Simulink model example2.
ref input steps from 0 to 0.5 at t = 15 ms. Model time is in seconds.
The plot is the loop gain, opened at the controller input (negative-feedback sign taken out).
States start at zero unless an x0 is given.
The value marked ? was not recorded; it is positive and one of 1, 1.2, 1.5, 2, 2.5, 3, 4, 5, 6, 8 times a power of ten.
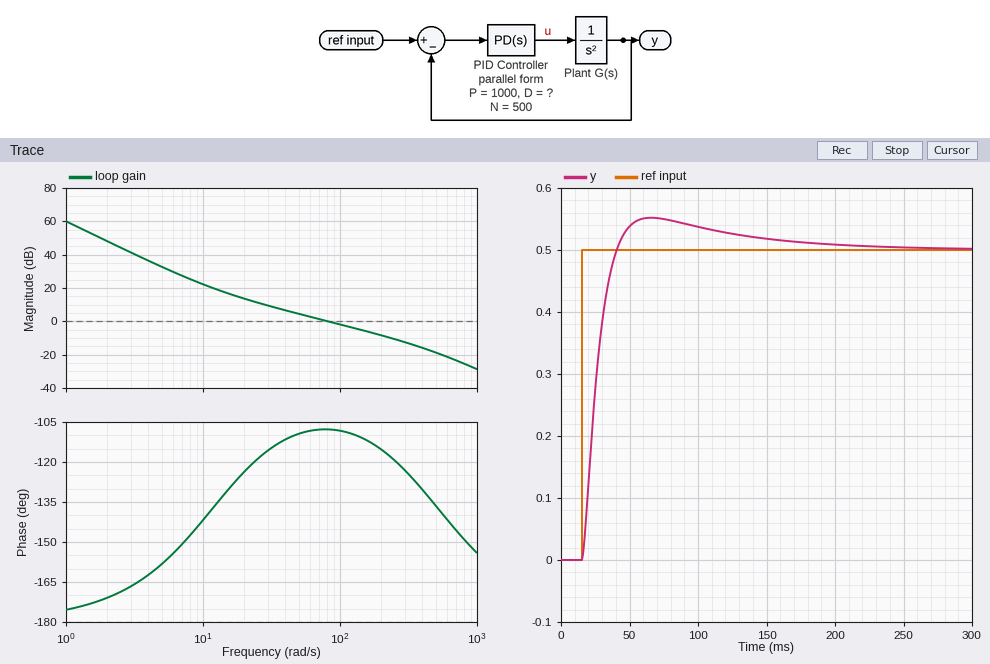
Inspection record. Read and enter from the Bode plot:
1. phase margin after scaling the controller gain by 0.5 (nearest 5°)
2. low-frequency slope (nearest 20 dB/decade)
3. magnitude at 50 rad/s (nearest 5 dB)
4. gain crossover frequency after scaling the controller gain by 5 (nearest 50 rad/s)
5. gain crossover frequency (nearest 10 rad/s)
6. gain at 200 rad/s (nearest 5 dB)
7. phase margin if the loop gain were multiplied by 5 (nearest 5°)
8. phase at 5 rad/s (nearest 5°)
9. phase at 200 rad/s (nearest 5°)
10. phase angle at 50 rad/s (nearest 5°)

70°
-40 dB/decade
5 dB
350 rad/s
80 rad/s
-10 dB
55°
-160°
-115°
-110°
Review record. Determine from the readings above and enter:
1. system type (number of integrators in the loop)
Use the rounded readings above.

2
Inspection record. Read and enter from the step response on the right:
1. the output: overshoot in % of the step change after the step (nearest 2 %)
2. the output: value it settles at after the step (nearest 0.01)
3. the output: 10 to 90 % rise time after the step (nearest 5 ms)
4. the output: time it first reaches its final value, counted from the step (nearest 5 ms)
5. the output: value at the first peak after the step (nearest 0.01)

10 %
0.50
15 ms
25 ms
0.55
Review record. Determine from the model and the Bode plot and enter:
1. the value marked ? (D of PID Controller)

80
